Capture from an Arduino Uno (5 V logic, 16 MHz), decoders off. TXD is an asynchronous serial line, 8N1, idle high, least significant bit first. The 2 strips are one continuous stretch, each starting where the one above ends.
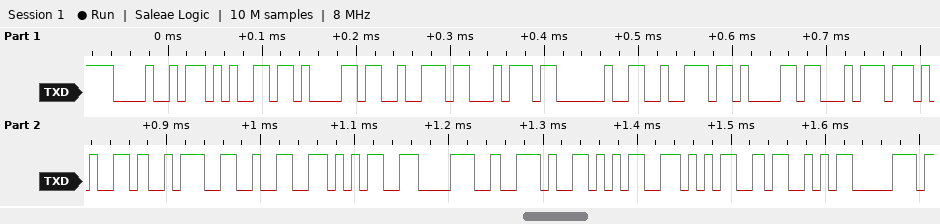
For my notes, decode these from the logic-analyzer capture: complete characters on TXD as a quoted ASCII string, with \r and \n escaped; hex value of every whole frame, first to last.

"Heart rate:258.55Sp"
48 65 61 72 74 20 72 61 74 65 3A 32 35 38 2E 35 35 53 70
